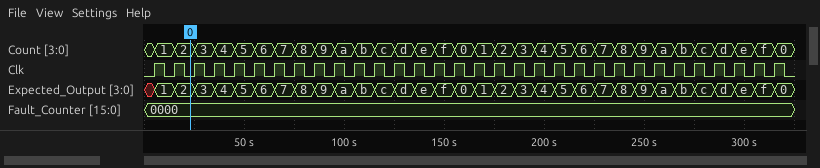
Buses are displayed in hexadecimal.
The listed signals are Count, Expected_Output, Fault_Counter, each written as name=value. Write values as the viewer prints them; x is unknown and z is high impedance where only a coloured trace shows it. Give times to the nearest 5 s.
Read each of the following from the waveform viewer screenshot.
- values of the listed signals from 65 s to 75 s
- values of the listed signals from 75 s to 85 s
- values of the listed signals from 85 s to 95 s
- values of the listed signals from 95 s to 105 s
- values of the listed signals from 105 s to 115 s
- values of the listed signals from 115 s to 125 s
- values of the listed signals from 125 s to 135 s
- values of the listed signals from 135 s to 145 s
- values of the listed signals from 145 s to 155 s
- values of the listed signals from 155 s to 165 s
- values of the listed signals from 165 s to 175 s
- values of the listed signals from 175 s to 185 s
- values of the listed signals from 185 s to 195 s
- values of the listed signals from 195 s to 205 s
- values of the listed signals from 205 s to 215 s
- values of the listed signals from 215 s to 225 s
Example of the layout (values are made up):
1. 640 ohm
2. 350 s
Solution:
1. Count=7, Expected_Output=7, Fault_Counter=0000
2. Count=8, Expected_Output=8, Fault_Counter=0000
3. Count=9, Expected_Output=9, Fault_Counter=0000
4. Count=a, Expected_Output=a, Fault_Counter=0000
5. Count=b, Expected_Output=b, Fault_Counter=0000
6. Count=c, Expected_Output=c, Fault_Counter=0000
7. Count=d, Expected_Output=d, Fault_Counter=0000
8. Count=e, Expected_Output=e, Fault_Counter=0000
9. Count=f, Expected_Output=f, Fault_Counter=0000
10. Count=0, Expected_Output=0, Fault_Counter=0000
11. Count=1, Expected_Output=1, Fault_Counter=0000
12. Count=2, Expected_Output=2, Fault_Counter=0000
13. Count=3, Expected_Output=3, Fault_Counter=0000
14. Count=4, Expected_Output=4, Fault_Counter=0000
15. Count=5, Expected_Output=5, Fault_Counter=0000
16. Count=6, Expected_Output=6, Fault_Counter=0000
